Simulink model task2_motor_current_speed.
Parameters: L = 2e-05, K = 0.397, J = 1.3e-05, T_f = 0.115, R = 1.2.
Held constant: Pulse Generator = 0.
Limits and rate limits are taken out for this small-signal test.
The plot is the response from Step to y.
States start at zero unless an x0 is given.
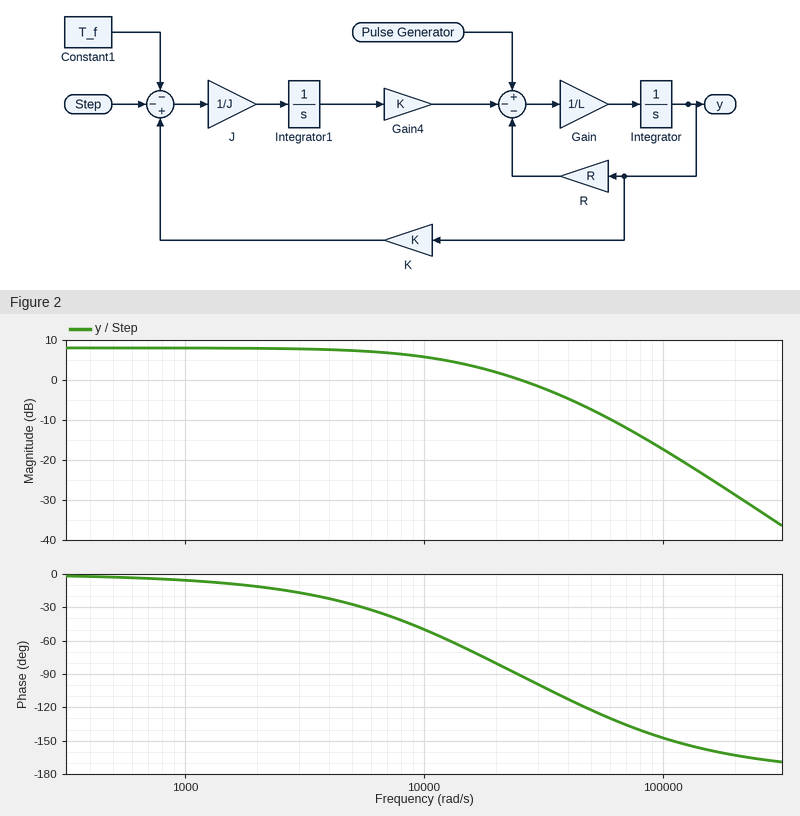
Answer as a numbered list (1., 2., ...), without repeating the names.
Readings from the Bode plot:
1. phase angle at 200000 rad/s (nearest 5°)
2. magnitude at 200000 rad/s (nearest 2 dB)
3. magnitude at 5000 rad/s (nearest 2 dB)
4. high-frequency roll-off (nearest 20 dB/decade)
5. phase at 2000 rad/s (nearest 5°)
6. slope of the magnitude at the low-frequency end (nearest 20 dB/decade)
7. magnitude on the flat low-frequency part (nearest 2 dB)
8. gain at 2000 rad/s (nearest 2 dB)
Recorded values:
1. -165°
2. -28 dB
3. 8 dB
4. -40 dB/decade
5. -10°
6. 0 dB/decade
7. 8 dB
8. 8 dB
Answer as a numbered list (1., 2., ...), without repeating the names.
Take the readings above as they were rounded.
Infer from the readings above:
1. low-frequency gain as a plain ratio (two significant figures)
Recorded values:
1. 2.5
